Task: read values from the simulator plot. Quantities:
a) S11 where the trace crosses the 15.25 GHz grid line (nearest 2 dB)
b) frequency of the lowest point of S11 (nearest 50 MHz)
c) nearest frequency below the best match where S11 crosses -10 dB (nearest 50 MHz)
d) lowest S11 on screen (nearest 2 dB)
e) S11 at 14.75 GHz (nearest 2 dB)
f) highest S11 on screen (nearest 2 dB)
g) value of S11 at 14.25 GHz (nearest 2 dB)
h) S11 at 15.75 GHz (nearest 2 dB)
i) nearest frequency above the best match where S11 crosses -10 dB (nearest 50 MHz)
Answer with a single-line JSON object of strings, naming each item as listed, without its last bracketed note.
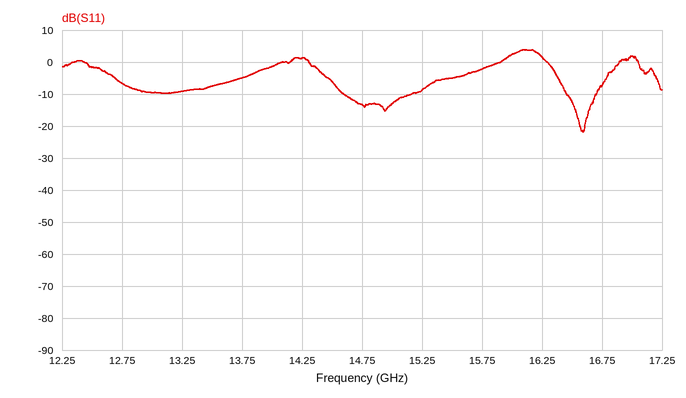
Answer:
{"S11 where the trace crosses the 15.25 GHz grid line": "-8 dB", "frequency of the lowest point of S11": "16.60 GHz", "nearest frequency below the best match where S11 crosses -10 dB": "16.45 GHz", "lowest S11 on screen": "-22 dB", "S11 at 14.75 GHz": "-14 dB", "highest S11 on screen": "4 dB", "value of S11 at 14.25 GHz": "2 dB", "S11 at 15.75 GHz": "-2 dB", "nearest frequency above the best match where S11 crosses -10 dB": "16.70 GHz"}
